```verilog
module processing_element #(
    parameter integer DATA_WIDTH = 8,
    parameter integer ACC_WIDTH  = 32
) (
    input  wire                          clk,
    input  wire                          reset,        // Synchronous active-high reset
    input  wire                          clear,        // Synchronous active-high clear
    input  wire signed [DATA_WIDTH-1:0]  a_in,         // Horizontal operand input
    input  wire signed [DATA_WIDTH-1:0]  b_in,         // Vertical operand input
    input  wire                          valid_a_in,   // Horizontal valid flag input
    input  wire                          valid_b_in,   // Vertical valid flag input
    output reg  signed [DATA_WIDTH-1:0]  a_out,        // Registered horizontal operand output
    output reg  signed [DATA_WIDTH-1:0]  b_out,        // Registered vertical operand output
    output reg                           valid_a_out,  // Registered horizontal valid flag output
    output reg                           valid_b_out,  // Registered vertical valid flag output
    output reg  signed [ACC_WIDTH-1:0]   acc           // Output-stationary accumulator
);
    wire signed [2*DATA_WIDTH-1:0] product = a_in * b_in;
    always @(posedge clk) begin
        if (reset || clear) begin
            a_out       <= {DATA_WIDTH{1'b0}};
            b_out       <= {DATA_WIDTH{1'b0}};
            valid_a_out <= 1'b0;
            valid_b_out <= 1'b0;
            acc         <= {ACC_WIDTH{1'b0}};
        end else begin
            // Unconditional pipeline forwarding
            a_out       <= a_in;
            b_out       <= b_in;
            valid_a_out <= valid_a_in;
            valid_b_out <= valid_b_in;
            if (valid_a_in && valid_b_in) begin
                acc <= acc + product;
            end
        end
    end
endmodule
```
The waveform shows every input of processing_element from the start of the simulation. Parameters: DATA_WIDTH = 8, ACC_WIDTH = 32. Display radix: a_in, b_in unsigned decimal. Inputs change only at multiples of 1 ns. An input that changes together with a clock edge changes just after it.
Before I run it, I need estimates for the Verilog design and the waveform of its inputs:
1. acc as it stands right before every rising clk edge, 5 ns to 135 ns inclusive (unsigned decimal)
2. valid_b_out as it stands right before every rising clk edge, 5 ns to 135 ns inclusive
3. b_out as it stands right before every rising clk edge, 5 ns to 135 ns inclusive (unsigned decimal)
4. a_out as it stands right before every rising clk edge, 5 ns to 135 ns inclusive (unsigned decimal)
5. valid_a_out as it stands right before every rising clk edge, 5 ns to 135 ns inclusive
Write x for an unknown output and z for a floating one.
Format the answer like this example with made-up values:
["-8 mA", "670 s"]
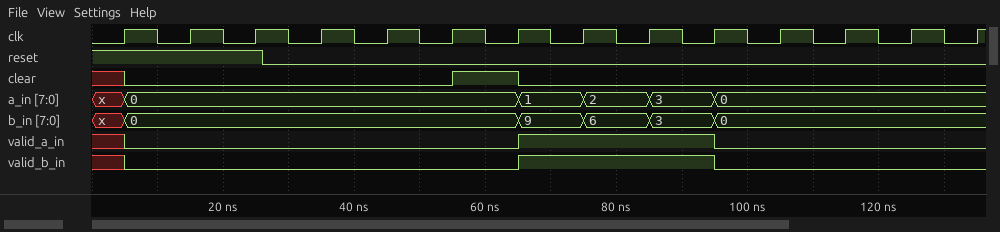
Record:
["x, 0, 0, 0, 0, 0, 0, 0, 9, 21, 30, 30, 30, 30", "x 0 0 0 0 0 0 0 1 1 1 0 0 0", "x, 0, 0, 0, 0, 0, 0, 0, 9, 6, 3, 0, 0, 0", "x, 0, 0, 0, 0, 0, 0, 0, 1, 2, 3, 0, 0, 0", "x 0 0 0 0 0 0 0 1 1 1 0 0 0"]
